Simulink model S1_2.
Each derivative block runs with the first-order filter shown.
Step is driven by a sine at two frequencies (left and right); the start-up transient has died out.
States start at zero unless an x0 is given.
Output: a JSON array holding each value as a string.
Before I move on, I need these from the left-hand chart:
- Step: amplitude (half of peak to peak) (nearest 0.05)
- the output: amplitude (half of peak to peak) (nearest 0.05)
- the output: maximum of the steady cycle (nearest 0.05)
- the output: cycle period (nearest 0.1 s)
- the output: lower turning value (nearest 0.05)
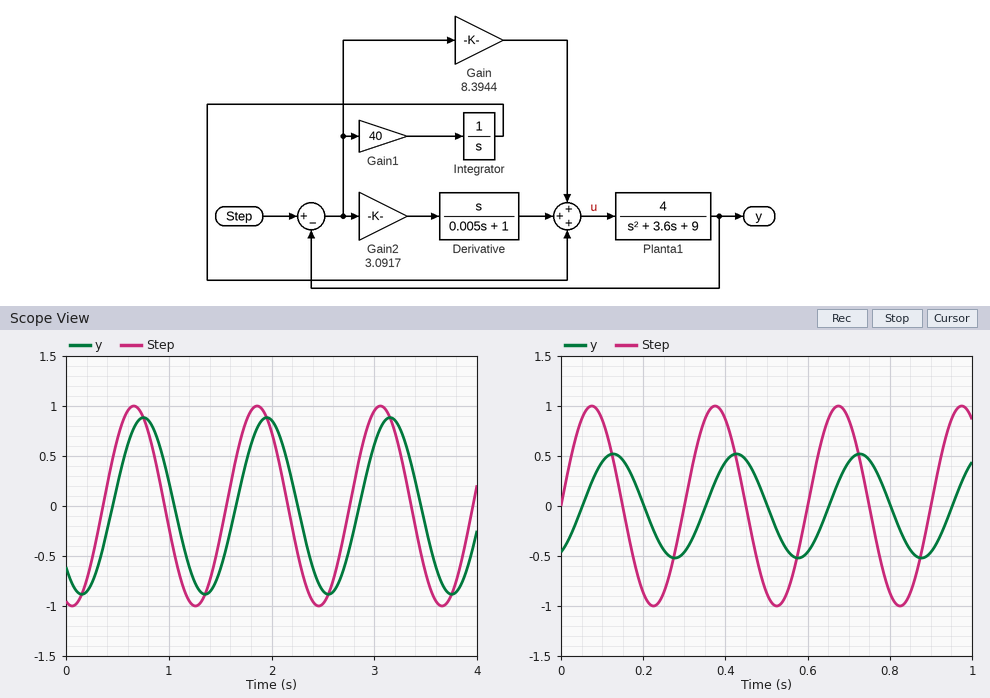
["1.00", "0.90", "0.90", "1.2 s", "-0.90"]
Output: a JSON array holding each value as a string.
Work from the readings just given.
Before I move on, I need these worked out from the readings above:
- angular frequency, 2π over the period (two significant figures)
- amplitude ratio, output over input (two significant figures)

["5.2 rad/s", "0.90"]
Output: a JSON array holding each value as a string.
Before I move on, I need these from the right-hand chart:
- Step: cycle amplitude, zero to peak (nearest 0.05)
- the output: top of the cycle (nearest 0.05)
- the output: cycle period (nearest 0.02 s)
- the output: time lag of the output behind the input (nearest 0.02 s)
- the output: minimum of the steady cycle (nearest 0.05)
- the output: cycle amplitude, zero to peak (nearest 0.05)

["1.00", "0.50", "0.30 s", "0.06 s", "-0.50", "0.50"]
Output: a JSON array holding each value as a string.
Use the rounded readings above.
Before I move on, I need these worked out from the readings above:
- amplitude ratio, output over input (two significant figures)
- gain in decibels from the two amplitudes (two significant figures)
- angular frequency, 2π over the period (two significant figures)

["0.50", "-6.0 dB", "21 rad/s"]
